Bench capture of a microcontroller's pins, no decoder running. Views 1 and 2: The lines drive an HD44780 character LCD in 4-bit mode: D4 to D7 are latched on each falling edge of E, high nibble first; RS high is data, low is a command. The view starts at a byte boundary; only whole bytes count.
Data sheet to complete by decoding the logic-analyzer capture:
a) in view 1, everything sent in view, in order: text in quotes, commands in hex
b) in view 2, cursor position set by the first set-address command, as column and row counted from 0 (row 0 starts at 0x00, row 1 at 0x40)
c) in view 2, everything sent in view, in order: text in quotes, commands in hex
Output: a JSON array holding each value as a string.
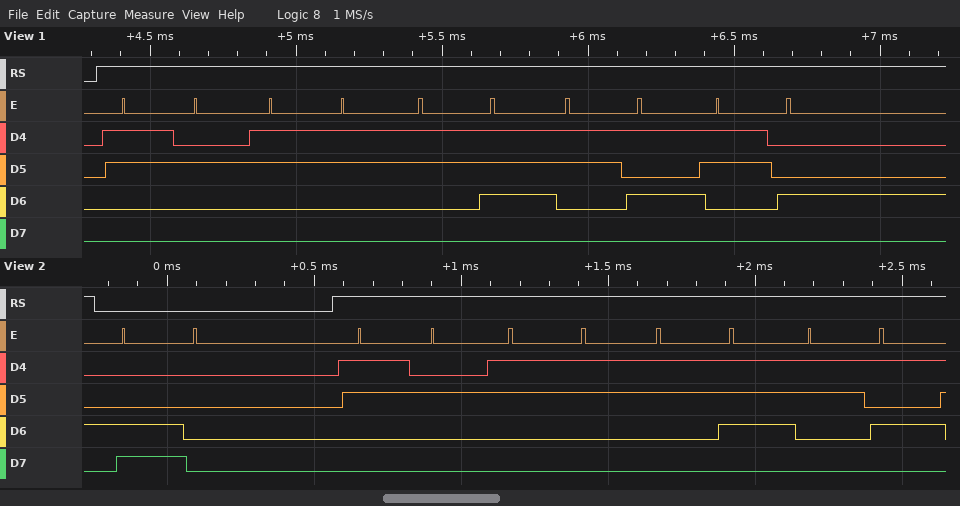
["\"23754\"", "column 0, row 1", "0xC0 \"2375\""]
